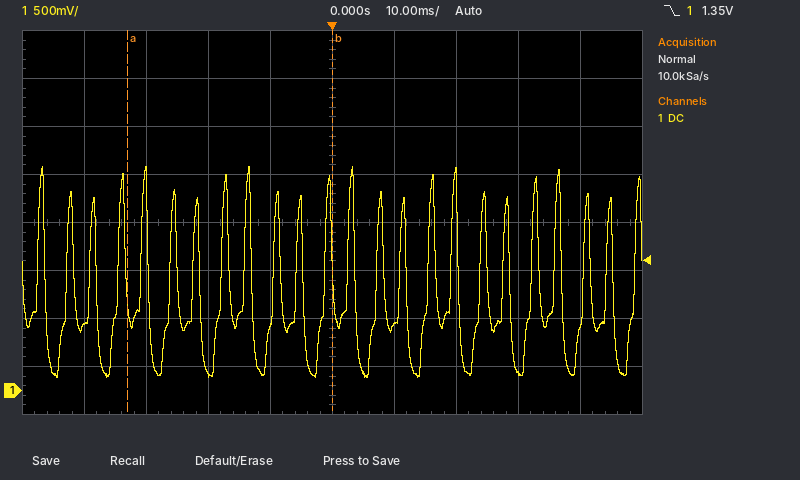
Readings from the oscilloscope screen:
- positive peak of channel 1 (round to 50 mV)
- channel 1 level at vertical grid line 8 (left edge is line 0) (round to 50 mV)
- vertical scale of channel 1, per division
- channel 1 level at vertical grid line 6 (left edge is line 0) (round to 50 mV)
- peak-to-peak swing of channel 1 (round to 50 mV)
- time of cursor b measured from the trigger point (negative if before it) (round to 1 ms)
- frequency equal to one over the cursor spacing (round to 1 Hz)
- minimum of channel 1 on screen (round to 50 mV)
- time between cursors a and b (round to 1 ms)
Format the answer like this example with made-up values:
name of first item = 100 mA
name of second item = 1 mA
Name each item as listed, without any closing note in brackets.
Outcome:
positive peak of channel 1 = 2.35 V
channel 1 level at vertical grid line 8 (left edge is line 0) = 200 mV
vertical scale of channel 1, per division = 500 mV
channel 1 level at vertical grid line 6 (left edge is line 0) = 650 mV
peak-to-peak swing of channel 1 = 2.20 V
time of cursor b measured from the trigger point (negative if before it) = 0 ms
frequency equal to one over the cursor spacing = 30 Hz
minimum of channel 1 on screen = 150 mV
time between cursors a and b = 33 ms
